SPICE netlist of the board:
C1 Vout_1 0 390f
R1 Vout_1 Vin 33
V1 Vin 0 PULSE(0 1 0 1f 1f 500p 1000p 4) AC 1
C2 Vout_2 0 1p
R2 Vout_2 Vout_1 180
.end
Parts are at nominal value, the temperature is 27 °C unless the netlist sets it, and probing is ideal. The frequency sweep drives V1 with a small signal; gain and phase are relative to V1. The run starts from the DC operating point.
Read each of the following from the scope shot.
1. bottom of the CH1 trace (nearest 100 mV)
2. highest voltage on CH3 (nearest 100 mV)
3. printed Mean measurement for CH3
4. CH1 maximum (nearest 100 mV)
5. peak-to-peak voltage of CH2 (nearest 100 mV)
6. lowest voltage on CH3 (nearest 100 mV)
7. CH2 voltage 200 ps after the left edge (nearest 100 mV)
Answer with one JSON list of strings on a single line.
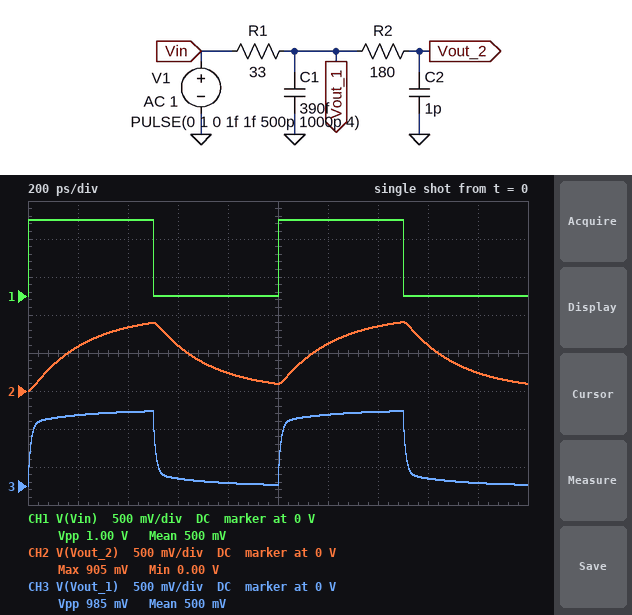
["0 V", "1.0 V", "500 mV", "1.0 V", "900 mV", "0 V", "600 mV"]
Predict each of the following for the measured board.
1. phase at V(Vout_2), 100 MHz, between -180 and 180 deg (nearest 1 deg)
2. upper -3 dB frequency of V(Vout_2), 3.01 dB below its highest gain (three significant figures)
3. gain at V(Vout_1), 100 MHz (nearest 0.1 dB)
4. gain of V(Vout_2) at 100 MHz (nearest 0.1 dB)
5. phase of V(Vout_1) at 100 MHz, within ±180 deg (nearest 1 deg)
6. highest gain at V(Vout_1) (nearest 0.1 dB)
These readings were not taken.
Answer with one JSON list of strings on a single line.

["-8 deg", "738 MHz", "0 dB", "-0.1 dB", "-2 deg", "0 dB"]
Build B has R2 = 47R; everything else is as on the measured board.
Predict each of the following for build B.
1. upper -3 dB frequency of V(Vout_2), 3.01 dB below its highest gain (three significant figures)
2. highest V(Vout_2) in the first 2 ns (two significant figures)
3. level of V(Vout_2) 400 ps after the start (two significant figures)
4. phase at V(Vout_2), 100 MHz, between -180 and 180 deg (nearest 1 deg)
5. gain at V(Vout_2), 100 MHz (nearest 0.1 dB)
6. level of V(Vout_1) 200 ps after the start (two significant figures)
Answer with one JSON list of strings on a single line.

["1.84 GHz", "1.0 V", "990 mV", "-3 deg", "0 dB", "950 mV"]
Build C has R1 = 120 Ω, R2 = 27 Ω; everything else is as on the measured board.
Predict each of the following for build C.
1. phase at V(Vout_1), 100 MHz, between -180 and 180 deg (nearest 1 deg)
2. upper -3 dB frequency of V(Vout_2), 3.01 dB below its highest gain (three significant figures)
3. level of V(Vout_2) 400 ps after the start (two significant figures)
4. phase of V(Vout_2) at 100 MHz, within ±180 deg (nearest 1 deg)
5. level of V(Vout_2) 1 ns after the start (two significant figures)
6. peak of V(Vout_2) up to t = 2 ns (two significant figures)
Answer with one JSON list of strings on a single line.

["-6 deg", "850 MHz", "880 mV", "-7 deg", "67 mV", "930 mV"]
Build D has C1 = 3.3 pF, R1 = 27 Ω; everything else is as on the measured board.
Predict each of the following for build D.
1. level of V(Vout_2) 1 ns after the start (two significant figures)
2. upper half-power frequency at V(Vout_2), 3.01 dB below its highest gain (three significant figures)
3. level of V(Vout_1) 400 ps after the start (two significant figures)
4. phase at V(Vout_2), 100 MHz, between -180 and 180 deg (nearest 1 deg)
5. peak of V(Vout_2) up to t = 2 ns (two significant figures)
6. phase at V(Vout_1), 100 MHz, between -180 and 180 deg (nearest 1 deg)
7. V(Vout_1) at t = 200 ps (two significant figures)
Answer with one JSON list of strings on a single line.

["140 mV", "650 MHz", "950 mV", "-11 deg", "860 mV", "-4 deg", "840 mV"]
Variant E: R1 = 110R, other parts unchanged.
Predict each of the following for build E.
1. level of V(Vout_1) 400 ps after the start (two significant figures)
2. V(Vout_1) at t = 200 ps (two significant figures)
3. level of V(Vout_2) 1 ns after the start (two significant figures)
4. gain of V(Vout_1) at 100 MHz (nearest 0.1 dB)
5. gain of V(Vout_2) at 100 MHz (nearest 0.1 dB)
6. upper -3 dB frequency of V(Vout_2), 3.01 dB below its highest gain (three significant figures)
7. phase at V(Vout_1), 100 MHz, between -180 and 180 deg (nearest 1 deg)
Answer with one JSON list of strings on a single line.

["880 mV", "760 mV", "170 mV", "-0.1 dB", "-0.2 dB", "514 MHz", "-5 deg"]
